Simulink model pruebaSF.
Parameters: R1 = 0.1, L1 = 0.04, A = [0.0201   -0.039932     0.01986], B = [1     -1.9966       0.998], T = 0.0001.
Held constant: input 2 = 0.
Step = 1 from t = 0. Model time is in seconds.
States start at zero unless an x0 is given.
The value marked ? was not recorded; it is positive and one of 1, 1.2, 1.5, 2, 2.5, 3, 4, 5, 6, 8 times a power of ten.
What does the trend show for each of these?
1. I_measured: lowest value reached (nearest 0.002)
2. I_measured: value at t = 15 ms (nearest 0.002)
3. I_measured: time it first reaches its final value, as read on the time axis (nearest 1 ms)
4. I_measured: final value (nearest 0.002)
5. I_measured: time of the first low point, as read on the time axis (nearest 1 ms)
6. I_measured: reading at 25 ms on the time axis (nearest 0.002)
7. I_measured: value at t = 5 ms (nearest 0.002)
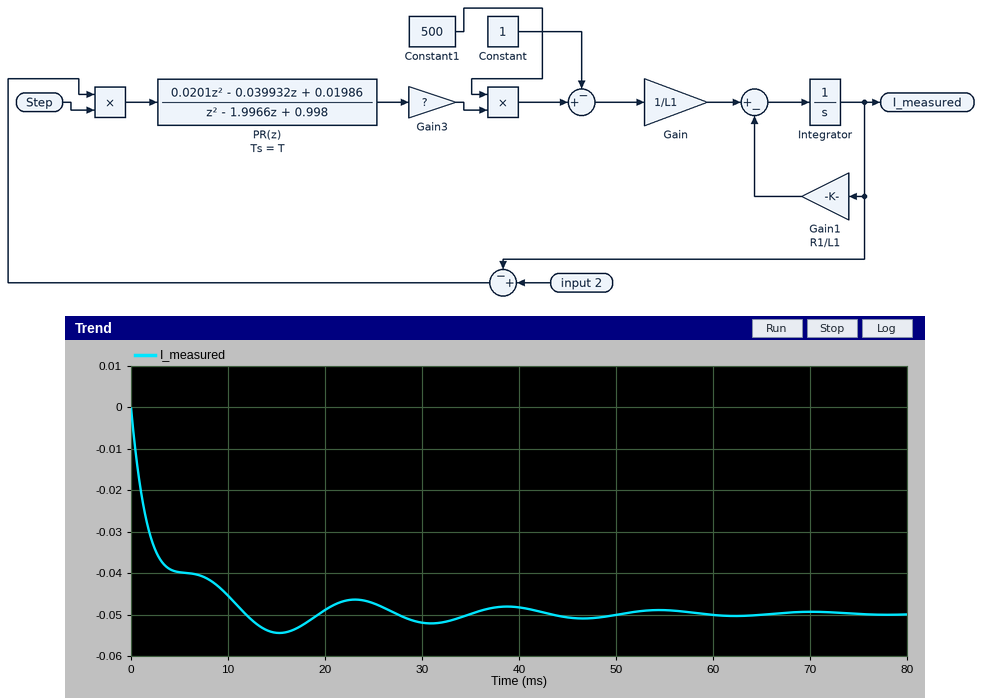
-0.054
-0.054
12 ms
-0.050
15 ms
-0.048
-0.040
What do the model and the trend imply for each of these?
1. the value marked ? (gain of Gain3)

2
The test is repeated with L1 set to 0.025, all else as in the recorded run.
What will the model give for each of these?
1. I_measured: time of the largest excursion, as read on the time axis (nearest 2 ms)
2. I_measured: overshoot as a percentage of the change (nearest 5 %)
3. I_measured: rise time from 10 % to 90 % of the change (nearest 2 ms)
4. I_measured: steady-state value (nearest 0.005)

14 ms
10 %
8 ms
-0.050
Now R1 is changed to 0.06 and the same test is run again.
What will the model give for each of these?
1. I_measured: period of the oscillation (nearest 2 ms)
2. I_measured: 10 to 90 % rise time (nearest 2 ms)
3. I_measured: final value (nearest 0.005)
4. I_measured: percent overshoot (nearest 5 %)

16 ms
10 ms
-0.050
10 %
